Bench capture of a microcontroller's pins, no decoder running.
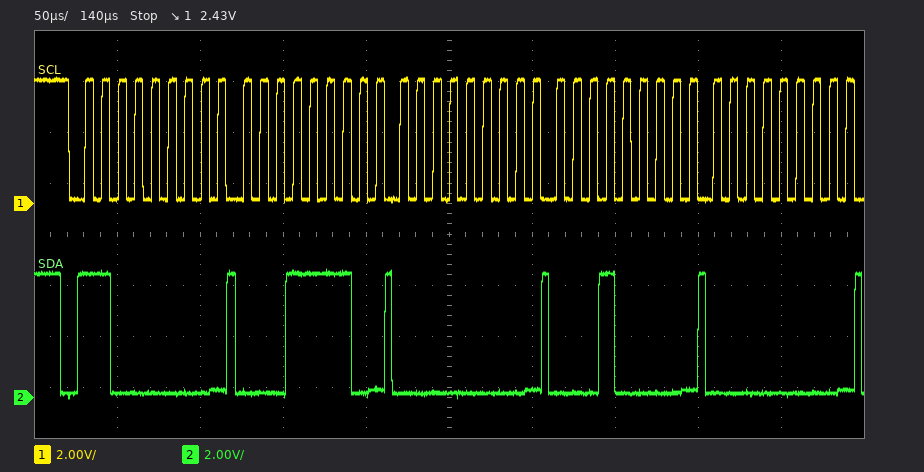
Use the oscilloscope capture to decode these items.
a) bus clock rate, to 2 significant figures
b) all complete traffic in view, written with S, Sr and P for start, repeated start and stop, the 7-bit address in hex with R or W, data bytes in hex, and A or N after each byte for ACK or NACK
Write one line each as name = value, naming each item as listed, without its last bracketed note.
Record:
bus clock rate, to 2 significant figures = 100 kHz
all complete traffic in view, written with S, Sr and P for start, repeated start and stop, the 7-bit address in hex with R or W, data bytes in hex, and A or N after each byte for ACK or NACK = S 60W A 1E A 00 A 10 A 00 A
